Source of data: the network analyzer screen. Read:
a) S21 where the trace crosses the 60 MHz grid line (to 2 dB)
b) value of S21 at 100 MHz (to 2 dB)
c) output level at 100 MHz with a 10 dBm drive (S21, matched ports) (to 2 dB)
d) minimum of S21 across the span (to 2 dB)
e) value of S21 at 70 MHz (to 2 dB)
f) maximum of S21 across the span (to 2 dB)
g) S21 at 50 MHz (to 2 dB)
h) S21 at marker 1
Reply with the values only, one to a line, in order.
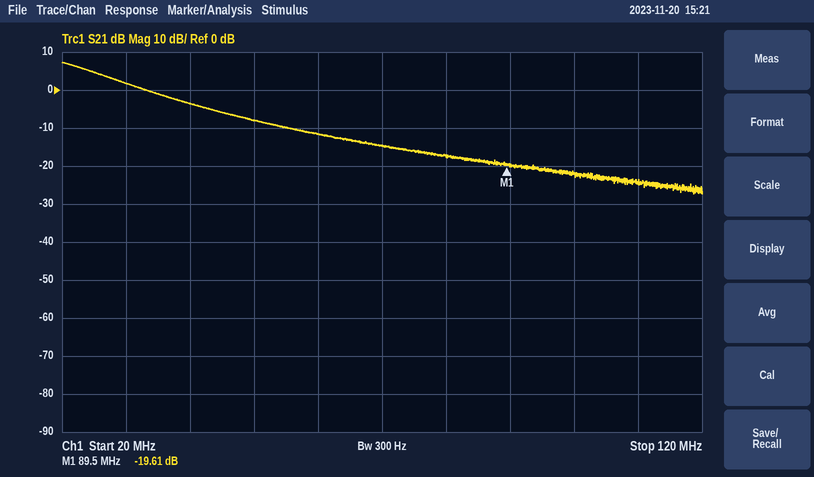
-12 dB
-22 dB
-12 dBm
-28 dB
-14 dB
8 dB
-8 dB
-19.61 dB
